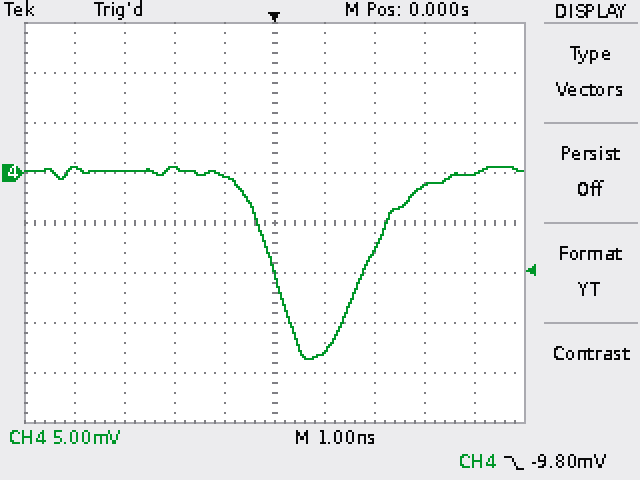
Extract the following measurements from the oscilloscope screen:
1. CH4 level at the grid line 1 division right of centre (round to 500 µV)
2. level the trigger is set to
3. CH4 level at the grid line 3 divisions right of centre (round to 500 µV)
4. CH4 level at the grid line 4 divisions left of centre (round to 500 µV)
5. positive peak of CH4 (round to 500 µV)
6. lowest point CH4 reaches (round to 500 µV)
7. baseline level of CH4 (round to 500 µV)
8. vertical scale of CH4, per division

-18.0 mV
-9.80 mV
-1.5 mV
500 µV
500 µV
-18.5 mV
0.0 mV
5 mV
